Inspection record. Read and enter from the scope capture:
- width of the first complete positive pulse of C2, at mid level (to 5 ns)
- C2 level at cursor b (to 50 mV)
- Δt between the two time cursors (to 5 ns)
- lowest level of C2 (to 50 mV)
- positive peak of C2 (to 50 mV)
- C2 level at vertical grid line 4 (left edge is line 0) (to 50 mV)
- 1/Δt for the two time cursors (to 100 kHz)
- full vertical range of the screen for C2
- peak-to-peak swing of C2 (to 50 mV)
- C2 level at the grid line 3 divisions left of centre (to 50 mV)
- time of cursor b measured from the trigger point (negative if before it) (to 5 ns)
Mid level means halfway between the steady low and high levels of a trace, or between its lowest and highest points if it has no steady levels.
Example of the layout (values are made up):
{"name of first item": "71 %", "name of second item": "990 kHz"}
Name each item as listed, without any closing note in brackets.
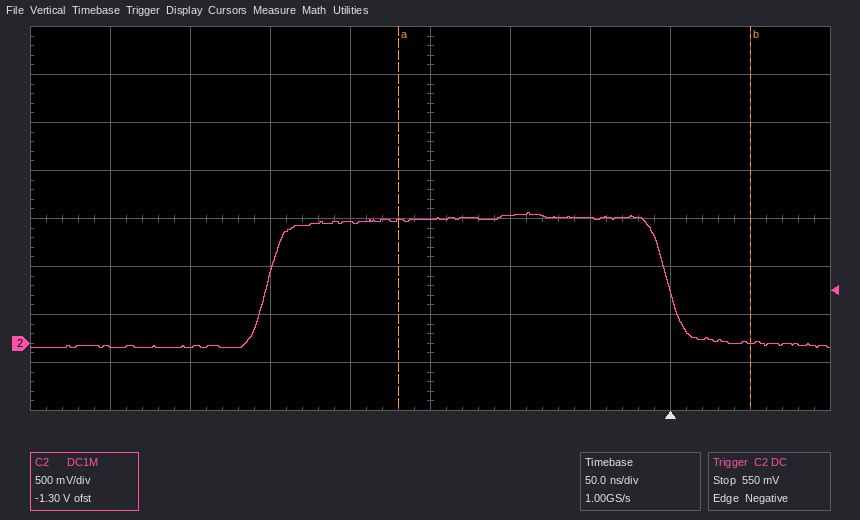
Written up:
{"width of the first complete positive pulse of C2, at mid level": "250 ns", "C2 level at cursor b": "0 mV", "Δt between the two time cursors": "220 ns", "lowest level of C2": "-50 mV", "positive peak of C2": "1.35 V", "C2 level at vertical grid line 4 (left edge is line 0)": "1.25 V", "1/Δt for the two time cursors": "4.5 MHz", "full vertical range of the screen for C2": "4 V", "peak-to-peak swing of C2": "1.40 V", "C2 level at the grid line 3 divisions left of centre": "-50 mV", "time of cursor b measured from the trigger point (negative if before it)": "+50 ns"}
